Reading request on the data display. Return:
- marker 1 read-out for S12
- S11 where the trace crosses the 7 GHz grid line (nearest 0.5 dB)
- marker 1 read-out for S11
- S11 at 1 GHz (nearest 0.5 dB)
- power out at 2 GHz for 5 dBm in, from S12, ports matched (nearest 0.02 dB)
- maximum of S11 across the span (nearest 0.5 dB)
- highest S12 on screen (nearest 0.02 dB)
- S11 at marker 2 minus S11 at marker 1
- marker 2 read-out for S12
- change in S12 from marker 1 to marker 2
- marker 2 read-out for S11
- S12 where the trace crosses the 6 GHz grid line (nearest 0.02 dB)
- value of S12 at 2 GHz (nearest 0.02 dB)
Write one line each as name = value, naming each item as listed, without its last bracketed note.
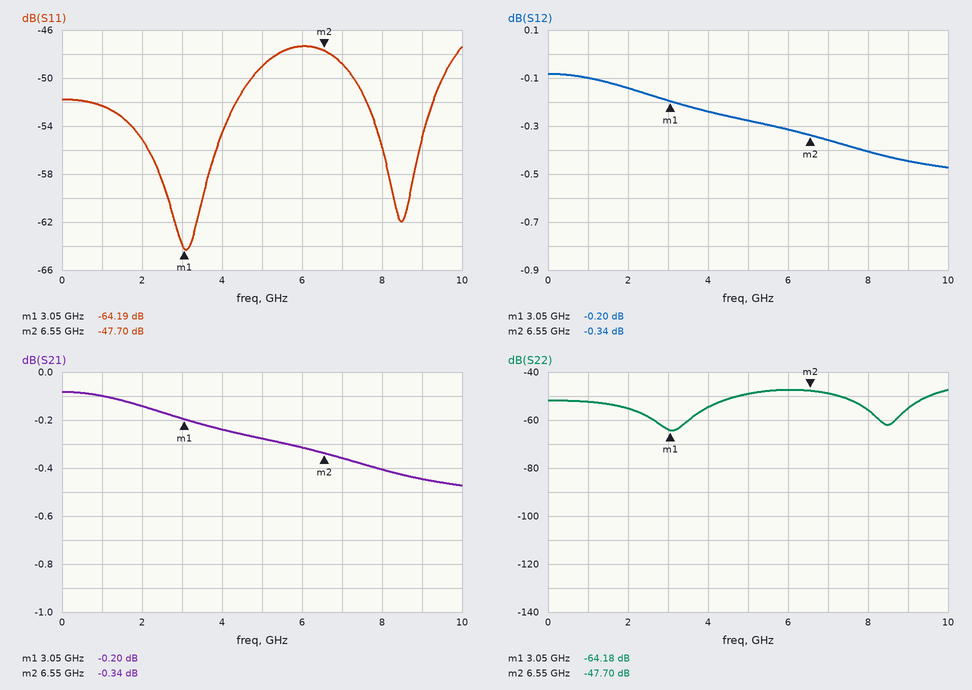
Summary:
marker 1 read-out for S12 = -0.20 dB
S11 where the trace crosses the 7 GHz grid line = -49.0 dB
marker 1 read-out for S11 = -64.19 dB
S11 at 1 GHz = -52.5 dB
power out at 2 GHz for 5 dBm in, from S12, ports matched = 4.86 dBm
maximum of S11 across the span = -47.5 dB
highest S12 on screen = -0.08 dB
S11 at marker 2 minus S11 at marker 1 = 16.49 dB
marker 2 read-out for S12 = -0.34 dB
change in S12 from marker 1 to marker 2 = -0.14 dB
marker 2 read-out for S11 = -47.70 dB
S12 where the trace crosses the 6 GHz grid line = -0.32 dB
value of S12 at 2 GHz = -0.14 dB
